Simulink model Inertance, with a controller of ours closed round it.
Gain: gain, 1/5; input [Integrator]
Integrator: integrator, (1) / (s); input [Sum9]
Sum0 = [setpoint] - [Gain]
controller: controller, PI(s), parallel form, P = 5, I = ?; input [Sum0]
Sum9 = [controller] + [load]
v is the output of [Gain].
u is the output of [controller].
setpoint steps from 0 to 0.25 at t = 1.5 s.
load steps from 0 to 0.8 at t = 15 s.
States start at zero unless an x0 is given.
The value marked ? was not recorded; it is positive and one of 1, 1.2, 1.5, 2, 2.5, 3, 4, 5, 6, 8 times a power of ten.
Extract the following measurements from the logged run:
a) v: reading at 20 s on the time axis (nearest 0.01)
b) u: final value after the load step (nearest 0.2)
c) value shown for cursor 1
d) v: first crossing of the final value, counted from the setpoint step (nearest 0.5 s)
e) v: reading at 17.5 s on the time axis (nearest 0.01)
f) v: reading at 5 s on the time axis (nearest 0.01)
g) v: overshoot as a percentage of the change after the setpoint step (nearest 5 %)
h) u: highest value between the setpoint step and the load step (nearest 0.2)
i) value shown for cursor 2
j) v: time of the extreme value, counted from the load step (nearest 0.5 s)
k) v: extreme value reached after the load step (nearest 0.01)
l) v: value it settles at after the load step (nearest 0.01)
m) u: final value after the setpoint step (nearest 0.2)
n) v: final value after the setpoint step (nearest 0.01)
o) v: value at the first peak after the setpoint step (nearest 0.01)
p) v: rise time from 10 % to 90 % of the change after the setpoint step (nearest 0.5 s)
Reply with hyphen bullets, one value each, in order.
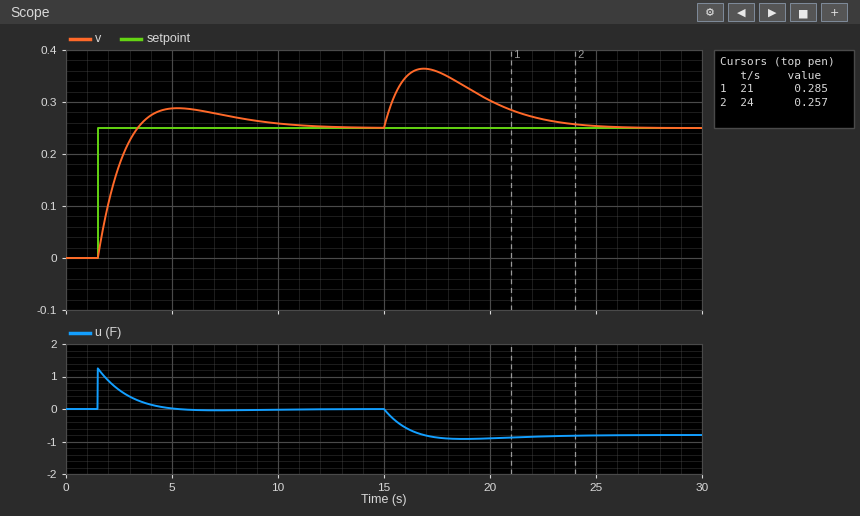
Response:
- 0.30
- -0.8
- 0.285
- 2.0 s
- 0.36
- 0.29
- 15 %
- 1.2
- 0.257
- 2.0 s
- 0.36
- 0.25
- 0.0
- 0.25
- 0.29
- 1.5 s
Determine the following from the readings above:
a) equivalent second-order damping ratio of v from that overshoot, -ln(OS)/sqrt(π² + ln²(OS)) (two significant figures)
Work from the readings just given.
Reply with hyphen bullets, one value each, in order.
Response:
- 0.52
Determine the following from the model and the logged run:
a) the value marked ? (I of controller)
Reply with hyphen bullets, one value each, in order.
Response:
- 1.5
